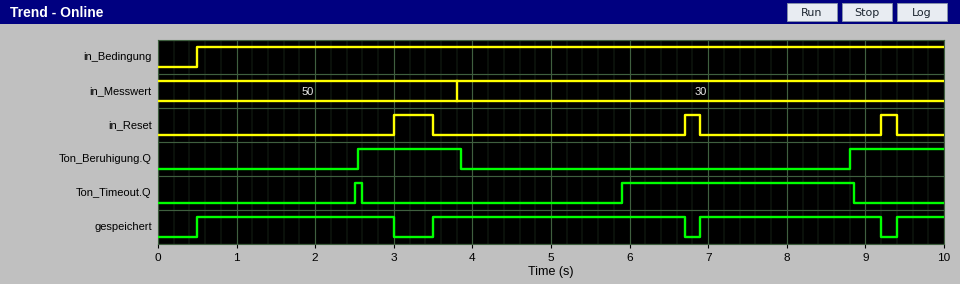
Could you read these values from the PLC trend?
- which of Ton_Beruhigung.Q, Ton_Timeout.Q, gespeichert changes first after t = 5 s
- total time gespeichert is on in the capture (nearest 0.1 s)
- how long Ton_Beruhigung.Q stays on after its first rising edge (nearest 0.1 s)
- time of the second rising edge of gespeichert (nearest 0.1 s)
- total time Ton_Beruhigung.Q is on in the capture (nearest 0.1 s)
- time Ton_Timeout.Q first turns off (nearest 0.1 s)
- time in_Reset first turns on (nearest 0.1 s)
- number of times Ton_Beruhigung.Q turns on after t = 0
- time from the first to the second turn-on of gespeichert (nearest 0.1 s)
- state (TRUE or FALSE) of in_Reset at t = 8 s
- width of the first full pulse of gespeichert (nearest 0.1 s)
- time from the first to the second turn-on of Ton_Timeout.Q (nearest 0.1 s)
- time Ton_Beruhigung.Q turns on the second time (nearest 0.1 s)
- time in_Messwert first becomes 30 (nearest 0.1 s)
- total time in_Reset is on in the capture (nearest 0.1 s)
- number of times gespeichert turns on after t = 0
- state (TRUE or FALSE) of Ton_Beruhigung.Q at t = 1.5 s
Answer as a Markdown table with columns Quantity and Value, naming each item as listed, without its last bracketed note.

| Quantity | Value |
|---|---|
| which of Ton_Beruhigung.Q, Ton_Timeout.Q, gespeichert changes first after t = 5 s | Ton_Timeout.Q |
| total time gespeichert is on in the capture | 8.6 s |
| how long Ton_Beruhigung.Q stays on after its first rising edge | 1.3 s |
| time of the second rising edge of gespeichert | 3.5 s |
| total time Ton_Beruhigung.Q is on in the capture | 2.5 s |
| time Ton_Timeout.Q first turns off | 2.6 s |
| time in_Reset first turns on | 3.0 s |
| number of times Ton_Beruhigung.Q turns on after t = 0 | 2 |
| time from the first to the second turn-on of gespeichert | 3.0 s |
| state (TRUE or FALSE) of in_Reset at t = 8 s | FALSE |
| width of the first full pulse of gespeichert | 2.5 s |
| time from the first to the second turn-on of Ton_Timeout.Q | 3.4 s |
| time Ton_Beruhigung.Q turns on the second time | 8.8 s |
| time in_Messwert first becomes 30 | 3.8 s |
| total time in_Reset is on in the capture | 0.9 s |
| number of times gespeichert turns on after t = 0 | 4 |
| state (TRUE or FALSE) of Ton_Beruhigung.Q at t = 1.5 s | FALSE |
